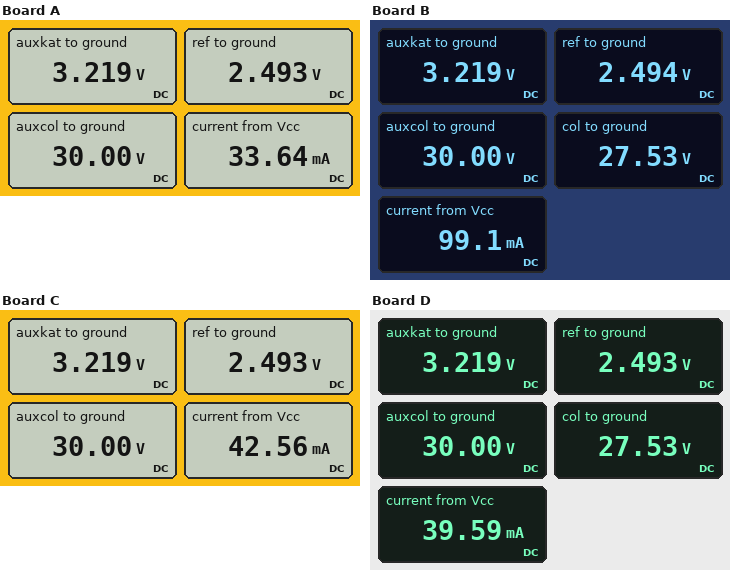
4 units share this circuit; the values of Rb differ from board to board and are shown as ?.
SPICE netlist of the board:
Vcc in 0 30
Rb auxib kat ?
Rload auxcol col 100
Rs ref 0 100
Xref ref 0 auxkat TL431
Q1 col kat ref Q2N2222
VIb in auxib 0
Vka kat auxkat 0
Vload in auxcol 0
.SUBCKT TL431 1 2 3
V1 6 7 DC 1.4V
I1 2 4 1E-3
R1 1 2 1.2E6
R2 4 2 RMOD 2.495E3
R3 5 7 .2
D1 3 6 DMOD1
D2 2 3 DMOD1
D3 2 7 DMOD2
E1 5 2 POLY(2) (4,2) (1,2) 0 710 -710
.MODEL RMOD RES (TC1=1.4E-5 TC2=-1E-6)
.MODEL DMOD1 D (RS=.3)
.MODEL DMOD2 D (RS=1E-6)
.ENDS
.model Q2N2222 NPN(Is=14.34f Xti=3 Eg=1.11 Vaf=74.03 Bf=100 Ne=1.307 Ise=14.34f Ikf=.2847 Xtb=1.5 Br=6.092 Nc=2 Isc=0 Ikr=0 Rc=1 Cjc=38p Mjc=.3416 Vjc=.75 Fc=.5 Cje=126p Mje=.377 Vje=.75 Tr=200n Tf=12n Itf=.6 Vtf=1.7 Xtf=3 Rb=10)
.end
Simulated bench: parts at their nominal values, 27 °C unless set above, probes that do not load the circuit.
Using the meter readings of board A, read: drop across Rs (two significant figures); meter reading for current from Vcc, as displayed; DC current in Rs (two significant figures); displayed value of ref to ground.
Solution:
2.5 V
33.64 mA
25 mA
2.493 V
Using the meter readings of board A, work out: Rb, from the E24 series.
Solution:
3 kΩ
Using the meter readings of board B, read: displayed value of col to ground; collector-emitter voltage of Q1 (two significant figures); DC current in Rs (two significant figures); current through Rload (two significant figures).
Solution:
27.53 V
25 V
25 mA
25 mA
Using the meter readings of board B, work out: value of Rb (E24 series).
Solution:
360 Ω
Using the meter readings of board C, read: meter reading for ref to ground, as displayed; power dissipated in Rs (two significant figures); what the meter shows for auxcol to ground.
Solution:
2.493 V
62 mW
30.00 V
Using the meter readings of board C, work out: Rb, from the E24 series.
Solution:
1.5 kΩ
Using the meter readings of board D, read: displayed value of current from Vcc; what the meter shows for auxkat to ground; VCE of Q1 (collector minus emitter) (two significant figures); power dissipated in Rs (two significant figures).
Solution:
39.59 mA
3.219 V
25 V
62 mW
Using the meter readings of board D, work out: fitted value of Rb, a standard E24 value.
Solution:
1.8 kΩ
